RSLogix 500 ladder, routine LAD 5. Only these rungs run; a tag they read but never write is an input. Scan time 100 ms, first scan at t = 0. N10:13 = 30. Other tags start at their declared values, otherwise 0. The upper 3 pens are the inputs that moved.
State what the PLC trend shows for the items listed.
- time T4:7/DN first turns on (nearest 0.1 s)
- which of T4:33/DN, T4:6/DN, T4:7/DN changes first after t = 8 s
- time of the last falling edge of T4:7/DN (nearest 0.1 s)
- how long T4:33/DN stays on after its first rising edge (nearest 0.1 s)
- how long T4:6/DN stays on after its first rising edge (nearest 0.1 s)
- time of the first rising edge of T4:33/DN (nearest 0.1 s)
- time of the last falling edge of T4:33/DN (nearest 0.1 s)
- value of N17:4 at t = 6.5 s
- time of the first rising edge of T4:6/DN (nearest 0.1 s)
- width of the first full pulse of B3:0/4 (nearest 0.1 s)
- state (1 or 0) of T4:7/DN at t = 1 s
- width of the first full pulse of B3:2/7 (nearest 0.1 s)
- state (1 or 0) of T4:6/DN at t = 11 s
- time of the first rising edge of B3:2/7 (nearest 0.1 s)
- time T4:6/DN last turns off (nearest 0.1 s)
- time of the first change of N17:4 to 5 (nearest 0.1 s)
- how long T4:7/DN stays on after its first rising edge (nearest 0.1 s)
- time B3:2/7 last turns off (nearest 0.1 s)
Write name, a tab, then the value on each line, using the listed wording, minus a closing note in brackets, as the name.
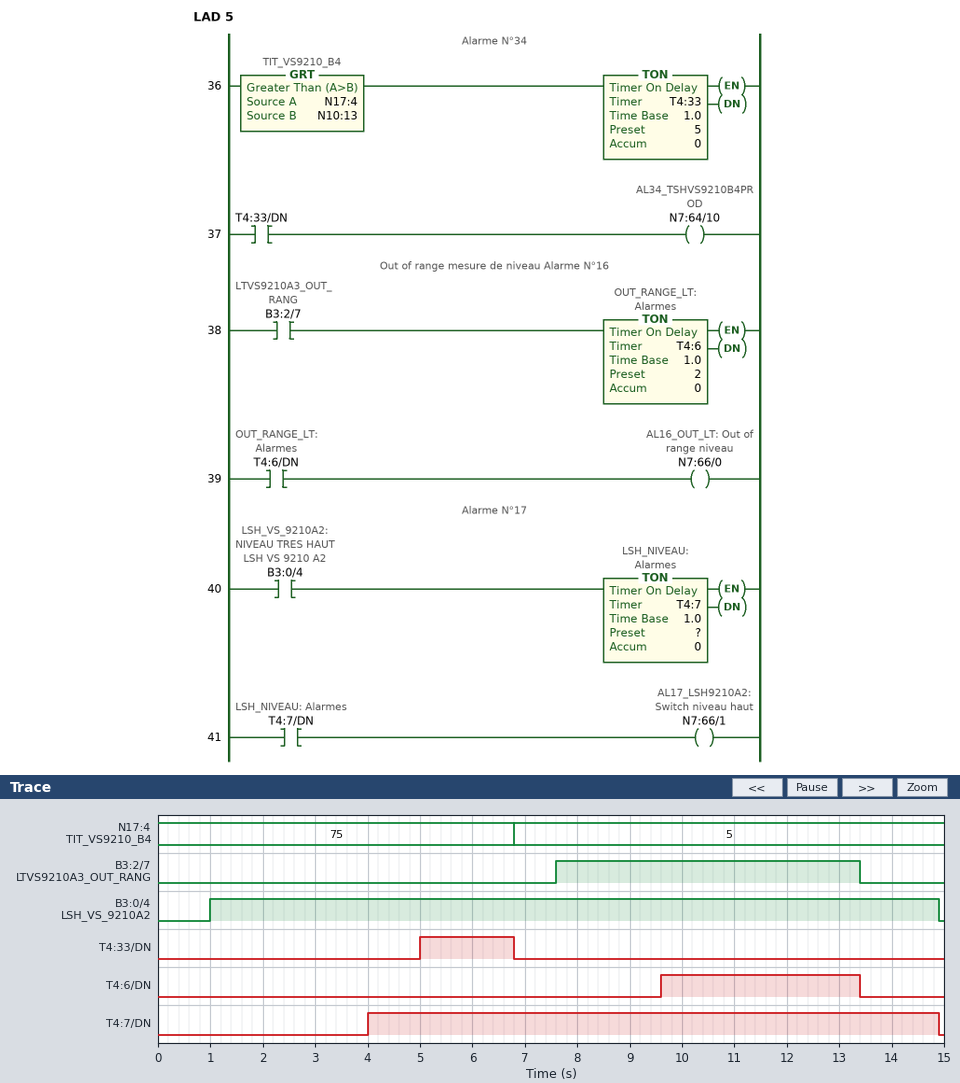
time T4:7/DN first turns on	4.0 s
which of T4:33/DN, T4:6/DN, T4:7/DN changes first after t = 8 s	T4:6/DN
time of the last falling edge of T4:7/DN	14.9 s
how long T4:33/DN stays on after its first rising edge	1.8 s
how long T4:6/DN stays on after its first rising edge	3.8 s
time of the first rising edge of T4:33/DN	5.0 s
time of the last falling edge of T4:33/DN	6.8 s
value of N17:4 at t = 6.5 s	75
time of the first rising edge of T4:6/DN	9.6 s
width of the first full pulse of B3:0/4	13.9 s
state (1 or 0) of T4:7/DN at t = 1 s	0
width of the first full pulse of B3:2/7	5.8 s
state (1 or 0) of T4:6/DN at t = 11 s	1
time of the first rising edge of B3:2/7	7.6 s
time T4:6/DN last turns off	13.4 s
time of the first change of N17:4 to 5	6.8 s
how long T4:7/DN stays on after its first rising edge	10.9 s
time B3:2/7 last turns off	13.4 s
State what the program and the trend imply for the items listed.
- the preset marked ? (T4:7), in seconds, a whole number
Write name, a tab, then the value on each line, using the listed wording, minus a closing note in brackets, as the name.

the preset marked ? (T4:7), in seconds, a whole number	3 s
